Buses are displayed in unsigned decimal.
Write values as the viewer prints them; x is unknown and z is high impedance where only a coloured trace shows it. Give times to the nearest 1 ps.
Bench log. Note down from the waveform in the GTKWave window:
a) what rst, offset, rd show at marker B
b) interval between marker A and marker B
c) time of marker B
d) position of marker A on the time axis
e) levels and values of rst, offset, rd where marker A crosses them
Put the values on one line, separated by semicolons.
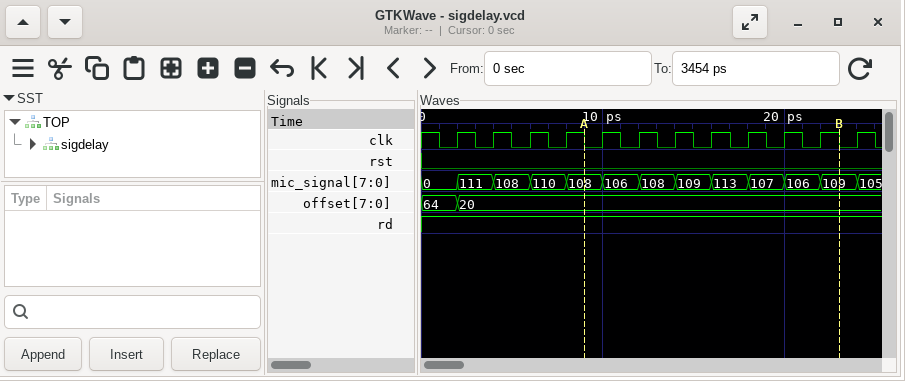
rst=0, offset=20, rd=1; 14 ps; 23 ps; 9 ps; rst=0, offset=20, rd=1
